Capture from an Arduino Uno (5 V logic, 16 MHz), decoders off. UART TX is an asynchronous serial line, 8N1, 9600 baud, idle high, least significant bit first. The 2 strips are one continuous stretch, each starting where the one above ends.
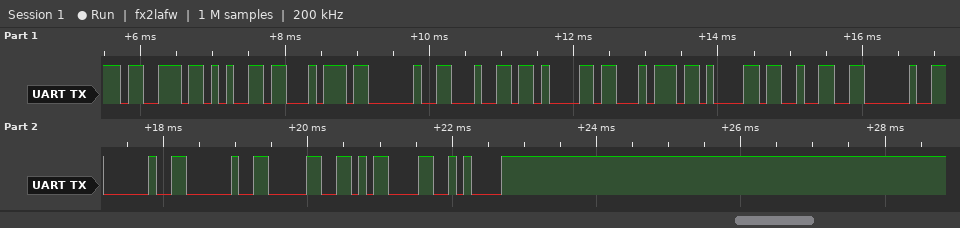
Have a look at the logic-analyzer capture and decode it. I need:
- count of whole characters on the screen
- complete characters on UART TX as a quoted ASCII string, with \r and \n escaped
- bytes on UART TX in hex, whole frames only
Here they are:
15
"set data2   0\r\n"
73 65 74 20 64 61 74 61 32 20 20 20 30 0D 0A
